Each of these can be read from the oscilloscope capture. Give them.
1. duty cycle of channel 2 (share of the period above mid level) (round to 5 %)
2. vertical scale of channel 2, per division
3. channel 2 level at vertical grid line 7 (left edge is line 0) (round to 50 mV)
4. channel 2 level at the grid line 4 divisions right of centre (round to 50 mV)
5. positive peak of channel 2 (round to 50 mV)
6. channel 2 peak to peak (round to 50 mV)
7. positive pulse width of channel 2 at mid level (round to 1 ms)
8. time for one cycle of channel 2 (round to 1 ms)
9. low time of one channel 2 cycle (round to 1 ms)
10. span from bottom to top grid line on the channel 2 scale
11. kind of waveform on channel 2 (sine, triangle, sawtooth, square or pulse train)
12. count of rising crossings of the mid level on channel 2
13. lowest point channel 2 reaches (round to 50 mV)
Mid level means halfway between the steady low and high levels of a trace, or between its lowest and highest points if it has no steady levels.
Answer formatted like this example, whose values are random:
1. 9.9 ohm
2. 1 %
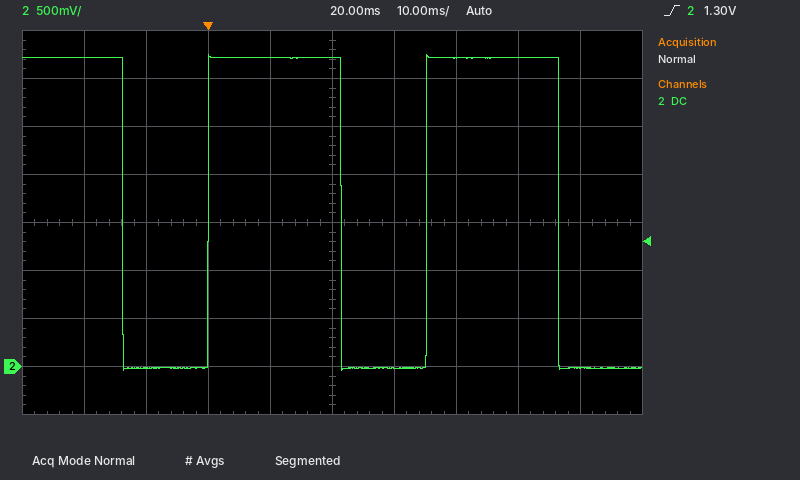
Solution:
1. 60 %
2. 500 mV
3. 3.20 V
4. 0 mV
5. 3.25 V
6. 3.30 V
7. 21 ms
8. 35 ms
9. 14 ms
10. 4 V
11. pulse train
12. 2
13. -50 mV
